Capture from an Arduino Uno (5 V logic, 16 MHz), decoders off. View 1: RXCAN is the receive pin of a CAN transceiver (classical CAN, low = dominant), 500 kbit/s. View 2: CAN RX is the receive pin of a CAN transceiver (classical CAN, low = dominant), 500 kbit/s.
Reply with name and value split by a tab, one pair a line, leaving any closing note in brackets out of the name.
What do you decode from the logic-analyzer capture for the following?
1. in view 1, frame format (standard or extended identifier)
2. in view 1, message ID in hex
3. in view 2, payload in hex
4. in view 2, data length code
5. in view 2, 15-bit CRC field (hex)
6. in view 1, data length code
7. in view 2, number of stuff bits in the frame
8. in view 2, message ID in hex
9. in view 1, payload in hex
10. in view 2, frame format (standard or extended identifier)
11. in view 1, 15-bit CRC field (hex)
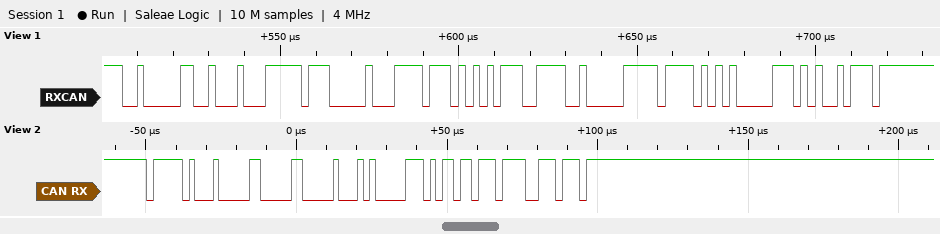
in view 1, frame format	standard
in view 1, message ID in hex	0x209
in view 2, payload in hex	10 0A 0D 6D
in view 2, data length code	4
in view 2, 15-bit CRC field	0x6F3B
in view 1, data length code	8
in view 2, number of stuff bits in the frame	5
in view 2, message ID in hex	0x7E2
in view 1, payload in hex	FF 00 F7 55 CF 20 FF 54
in view 2, frame format	standard
in view 1, 15-bit CRC field	0x0D4B
